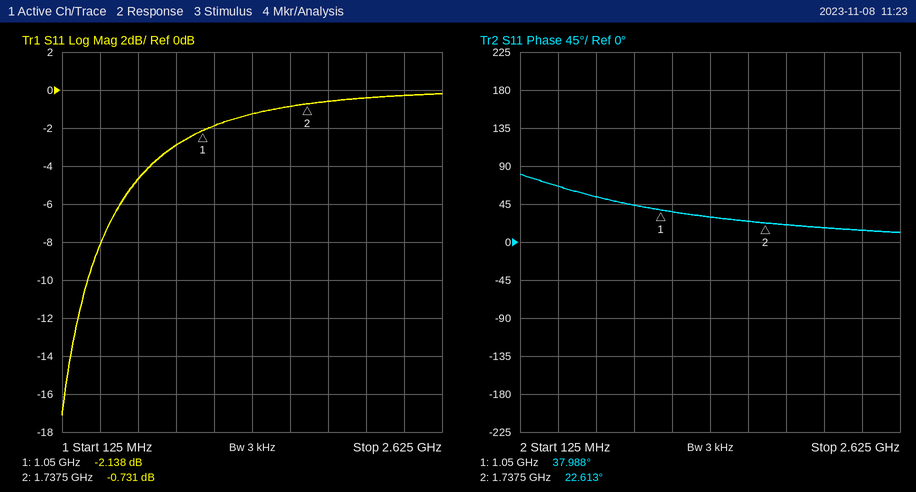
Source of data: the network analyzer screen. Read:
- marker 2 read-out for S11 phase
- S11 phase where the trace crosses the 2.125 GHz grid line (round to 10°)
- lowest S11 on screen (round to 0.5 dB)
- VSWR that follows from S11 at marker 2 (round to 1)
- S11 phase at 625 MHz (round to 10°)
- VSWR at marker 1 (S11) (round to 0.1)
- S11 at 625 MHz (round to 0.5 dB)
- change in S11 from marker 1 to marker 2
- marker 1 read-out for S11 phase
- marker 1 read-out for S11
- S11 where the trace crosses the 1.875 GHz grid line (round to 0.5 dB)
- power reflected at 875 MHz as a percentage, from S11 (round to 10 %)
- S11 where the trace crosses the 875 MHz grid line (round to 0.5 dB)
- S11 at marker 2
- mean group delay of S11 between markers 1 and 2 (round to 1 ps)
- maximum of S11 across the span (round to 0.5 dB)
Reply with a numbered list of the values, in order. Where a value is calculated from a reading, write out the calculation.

1. 22.613°
2. 20°
3. -17.0 dB
4. (1 + 0.9193)/(1 − 0.9193) ≈ 24
5. 50°
6. (1 + 0.7818)/(1 − 0.7818) ≈ 8.2
7. -4.5 dB
8. -0.731 − (-2.138) = 1.407 dB
9. 37.988°
10. -2.138 dB
11. -0.5 dB
12. 10^(-3/10) ≈ 50 %
13. -3.0 dB
14. -0.731 dB
15. −(22.613° − (37.988°))/(360° × 687.5 MHz) ≈ 62 ps
16. 0.0 dB
